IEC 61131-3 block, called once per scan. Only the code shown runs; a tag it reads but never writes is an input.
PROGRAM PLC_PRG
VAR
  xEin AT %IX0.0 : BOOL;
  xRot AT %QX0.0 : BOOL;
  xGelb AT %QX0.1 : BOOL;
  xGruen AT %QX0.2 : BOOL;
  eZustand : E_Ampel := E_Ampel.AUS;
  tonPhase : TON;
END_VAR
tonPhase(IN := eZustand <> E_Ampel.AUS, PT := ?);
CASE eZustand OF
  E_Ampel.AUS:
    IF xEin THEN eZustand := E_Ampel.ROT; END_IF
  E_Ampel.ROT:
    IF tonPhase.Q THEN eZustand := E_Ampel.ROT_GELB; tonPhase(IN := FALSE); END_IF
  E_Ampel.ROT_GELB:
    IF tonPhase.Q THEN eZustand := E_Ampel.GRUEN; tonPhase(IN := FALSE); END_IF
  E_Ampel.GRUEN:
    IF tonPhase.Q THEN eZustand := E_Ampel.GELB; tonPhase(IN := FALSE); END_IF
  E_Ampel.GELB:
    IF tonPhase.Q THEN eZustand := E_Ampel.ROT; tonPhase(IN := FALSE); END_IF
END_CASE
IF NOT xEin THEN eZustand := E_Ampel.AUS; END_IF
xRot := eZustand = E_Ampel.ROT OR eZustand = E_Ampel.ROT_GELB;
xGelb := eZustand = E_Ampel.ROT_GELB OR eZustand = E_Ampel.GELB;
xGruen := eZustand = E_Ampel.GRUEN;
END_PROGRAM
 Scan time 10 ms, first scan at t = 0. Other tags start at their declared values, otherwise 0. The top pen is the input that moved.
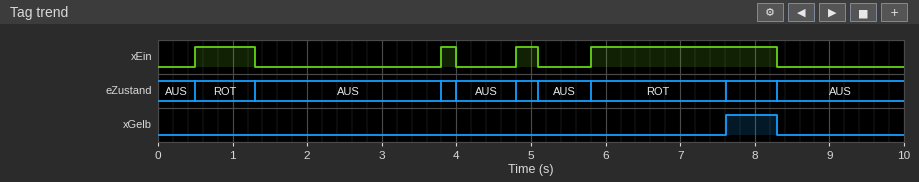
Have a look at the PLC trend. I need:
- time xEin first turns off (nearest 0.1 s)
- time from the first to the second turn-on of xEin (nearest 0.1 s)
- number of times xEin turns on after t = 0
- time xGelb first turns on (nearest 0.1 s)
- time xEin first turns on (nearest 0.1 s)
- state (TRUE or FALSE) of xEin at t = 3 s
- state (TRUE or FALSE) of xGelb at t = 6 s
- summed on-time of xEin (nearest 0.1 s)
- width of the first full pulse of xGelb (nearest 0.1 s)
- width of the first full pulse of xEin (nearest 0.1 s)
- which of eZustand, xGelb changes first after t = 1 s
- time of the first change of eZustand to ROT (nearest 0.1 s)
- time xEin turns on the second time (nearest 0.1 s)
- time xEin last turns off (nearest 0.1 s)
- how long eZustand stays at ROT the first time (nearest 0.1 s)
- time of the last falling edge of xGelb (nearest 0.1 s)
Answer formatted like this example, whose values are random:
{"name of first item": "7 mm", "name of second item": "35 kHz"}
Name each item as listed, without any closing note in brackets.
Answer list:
{"time xEin first turns off": "1.3 s", "time from the first to the second turn-on of xEin": "3.3 s", "number of times xEin turns on after t = 0": "4", "time xGelb first turns on": "7.6 s", "time xEin first turns on": "0.5 s", "state (TRUE or FALSE) of xEin at t = 3 s": "FALSE", "state (TRUE or FALSE) of xGelb at t = 6 s": "FALSE", "summed on-time of xEin": "3.8 s", "width of the first full pulse of xGelb": "0.7 s", "width of the first full pulse of xEin": "0.8 s", "which of eZustand, xGelb changes first after t = 1 s": "eZustand", "time of the first change of eZustand to ROT": "0.5 s", "time xEin turns on the second time": "3.8 s", "time xEin last turns off": "8.3 s", "how long eZustand stays at ROT the first time": "0.8 s", "time of the last falling edge of xGelb": "8.3 s"}
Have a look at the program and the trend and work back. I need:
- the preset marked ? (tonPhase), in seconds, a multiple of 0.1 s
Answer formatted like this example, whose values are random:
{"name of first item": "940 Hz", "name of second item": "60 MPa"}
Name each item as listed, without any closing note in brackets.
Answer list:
{"the preset marked ? (tonPhase), in seconds, a multiple of 0.1 s": "1.8 s"}
